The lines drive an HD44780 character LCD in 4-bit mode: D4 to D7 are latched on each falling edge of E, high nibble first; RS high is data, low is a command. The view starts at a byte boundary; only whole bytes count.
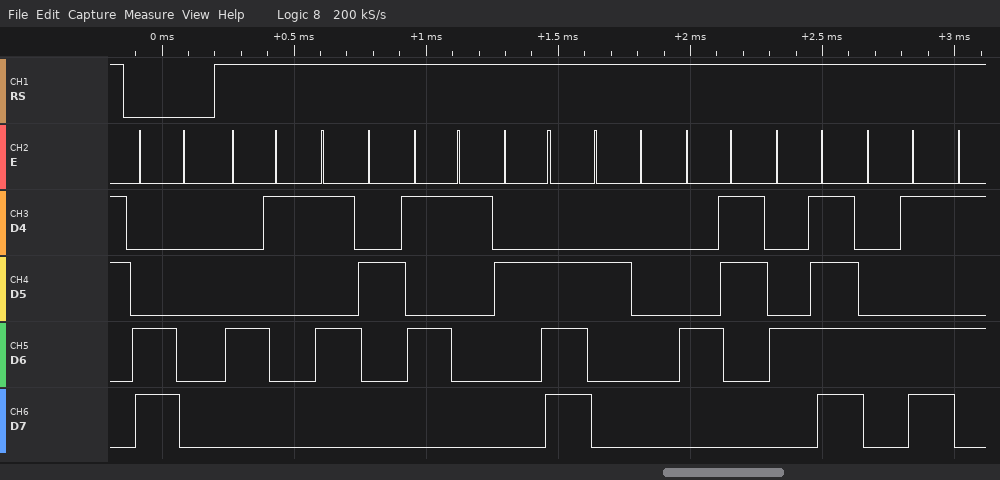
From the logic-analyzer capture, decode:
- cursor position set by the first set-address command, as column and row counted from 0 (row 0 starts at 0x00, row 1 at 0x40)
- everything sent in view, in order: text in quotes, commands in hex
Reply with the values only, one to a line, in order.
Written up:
column 0, row 1
0xC0 "ARQ. COM"
